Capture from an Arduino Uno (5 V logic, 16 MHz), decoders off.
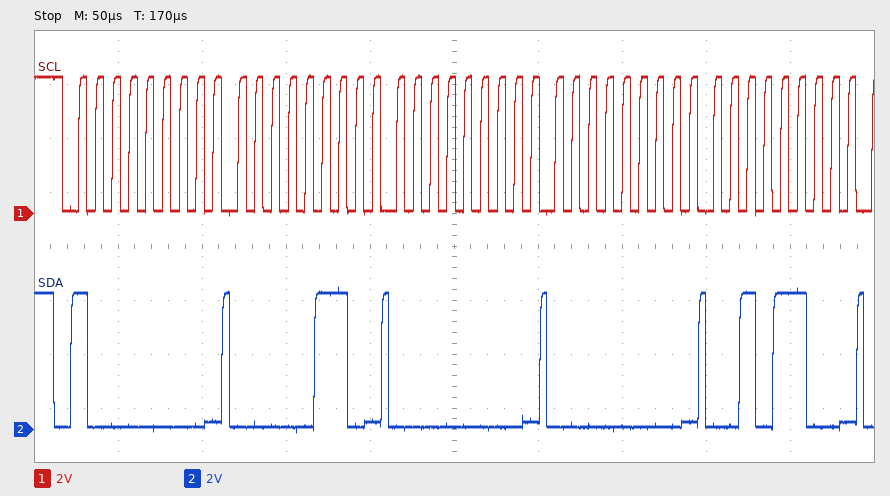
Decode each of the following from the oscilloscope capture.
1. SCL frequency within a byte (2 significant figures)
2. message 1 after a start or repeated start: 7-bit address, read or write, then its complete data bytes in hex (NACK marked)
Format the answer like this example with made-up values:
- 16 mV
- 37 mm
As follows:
- 100 kHz
- 0x40 write: 06 00 00 2C
